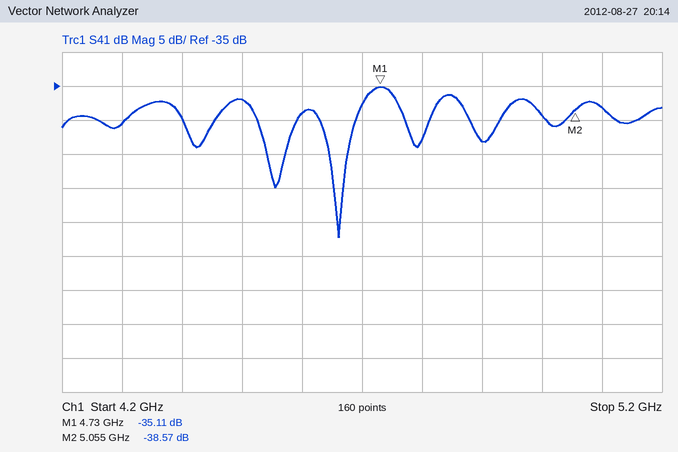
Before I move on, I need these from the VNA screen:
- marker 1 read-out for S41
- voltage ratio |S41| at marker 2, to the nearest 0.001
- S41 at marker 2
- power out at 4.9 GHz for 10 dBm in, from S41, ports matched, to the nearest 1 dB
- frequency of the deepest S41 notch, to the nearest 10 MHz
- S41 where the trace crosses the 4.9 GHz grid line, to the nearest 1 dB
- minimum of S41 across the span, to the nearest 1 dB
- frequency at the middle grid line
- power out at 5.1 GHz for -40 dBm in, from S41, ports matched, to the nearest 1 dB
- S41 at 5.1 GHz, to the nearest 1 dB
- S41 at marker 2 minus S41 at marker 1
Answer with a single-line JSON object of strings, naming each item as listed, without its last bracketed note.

{"marker 1 read-out for S41": "-35.11 dB", "voltage ratio |S41| at marker 2, to the nearest 0.001": "0.012", "S41 at marker 2": "-38.57 dB", "power out at 4.9 GHz for 10 dBm in, from S41, ports matched, to the nearest 1 dB": "-33 dBm", "frequency of the deepest S41 notch, to the nearest 10 MHz": "4.66 GHz", "S41 where the trace crosses the 4.9 GHz grid line, to the nearest 1 dB": "-43 dB", "minimum of S41 across the span, to the nearest 1 dB": "-57 dB", "frequency at the middle grid line": "4.7 GHz", "power out at 5.1 GHz for -40 dBm in, from S41, ports matched, to the nearest 1 dB": "-78 dBm", "S41 at 5.1 GHz, to the nearest 1 dB": "-38 dB", "S41 at marker 2 minus S41 at marker 1": "-3.46 dB"}
